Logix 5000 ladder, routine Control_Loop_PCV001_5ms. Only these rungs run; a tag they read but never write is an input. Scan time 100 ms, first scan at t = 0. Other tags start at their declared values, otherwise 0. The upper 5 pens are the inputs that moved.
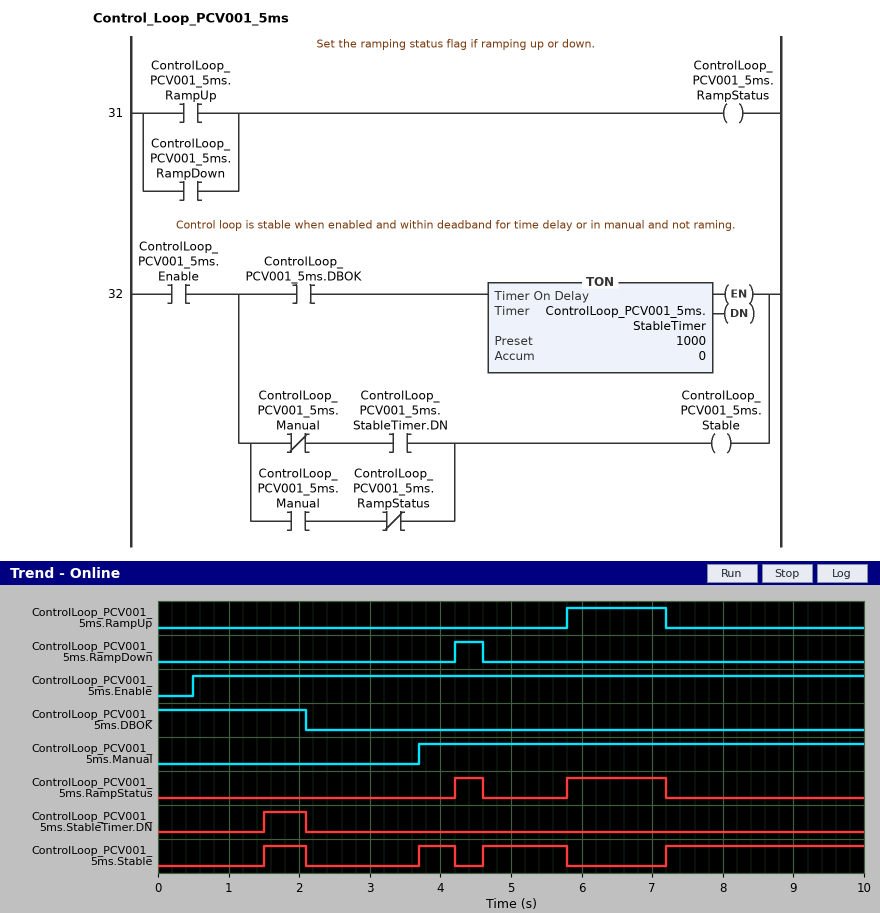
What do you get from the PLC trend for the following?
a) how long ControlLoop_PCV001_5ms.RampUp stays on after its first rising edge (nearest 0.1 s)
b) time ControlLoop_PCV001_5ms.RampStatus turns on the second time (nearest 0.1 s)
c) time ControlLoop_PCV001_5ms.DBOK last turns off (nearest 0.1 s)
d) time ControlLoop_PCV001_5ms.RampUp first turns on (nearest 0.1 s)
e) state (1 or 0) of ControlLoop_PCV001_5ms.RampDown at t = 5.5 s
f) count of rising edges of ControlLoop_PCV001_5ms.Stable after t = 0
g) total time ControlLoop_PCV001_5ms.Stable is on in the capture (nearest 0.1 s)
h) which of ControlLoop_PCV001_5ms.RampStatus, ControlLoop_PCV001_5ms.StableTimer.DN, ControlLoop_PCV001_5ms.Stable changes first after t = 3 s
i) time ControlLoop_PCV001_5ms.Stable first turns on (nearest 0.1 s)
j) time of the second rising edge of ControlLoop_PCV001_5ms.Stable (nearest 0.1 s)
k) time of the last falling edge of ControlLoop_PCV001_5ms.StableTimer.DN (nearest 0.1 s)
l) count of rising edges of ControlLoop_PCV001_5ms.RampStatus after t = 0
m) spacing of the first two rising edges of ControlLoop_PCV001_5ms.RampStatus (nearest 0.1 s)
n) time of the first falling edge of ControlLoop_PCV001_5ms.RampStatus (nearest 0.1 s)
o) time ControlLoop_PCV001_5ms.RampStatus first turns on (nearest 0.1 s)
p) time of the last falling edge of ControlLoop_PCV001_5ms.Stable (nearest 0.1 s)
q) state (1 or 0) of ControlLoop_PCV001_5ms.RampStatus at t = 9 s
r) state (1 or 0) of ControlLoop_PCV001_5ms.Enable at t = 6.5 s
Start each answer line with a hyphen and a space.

- 1.4 s
- 5.8 s
- 2.1 s
- 5.8 s
- 0
- 4
- 5.1 s
- ControlLoop_PCV001_5ms.Stable
- 1.5 s
- 3.7 s
- 2.1 s
- 2
- 1.6 s
- 4.6 s
- 4.2 s
- 5.8 s
- 0
- 1
